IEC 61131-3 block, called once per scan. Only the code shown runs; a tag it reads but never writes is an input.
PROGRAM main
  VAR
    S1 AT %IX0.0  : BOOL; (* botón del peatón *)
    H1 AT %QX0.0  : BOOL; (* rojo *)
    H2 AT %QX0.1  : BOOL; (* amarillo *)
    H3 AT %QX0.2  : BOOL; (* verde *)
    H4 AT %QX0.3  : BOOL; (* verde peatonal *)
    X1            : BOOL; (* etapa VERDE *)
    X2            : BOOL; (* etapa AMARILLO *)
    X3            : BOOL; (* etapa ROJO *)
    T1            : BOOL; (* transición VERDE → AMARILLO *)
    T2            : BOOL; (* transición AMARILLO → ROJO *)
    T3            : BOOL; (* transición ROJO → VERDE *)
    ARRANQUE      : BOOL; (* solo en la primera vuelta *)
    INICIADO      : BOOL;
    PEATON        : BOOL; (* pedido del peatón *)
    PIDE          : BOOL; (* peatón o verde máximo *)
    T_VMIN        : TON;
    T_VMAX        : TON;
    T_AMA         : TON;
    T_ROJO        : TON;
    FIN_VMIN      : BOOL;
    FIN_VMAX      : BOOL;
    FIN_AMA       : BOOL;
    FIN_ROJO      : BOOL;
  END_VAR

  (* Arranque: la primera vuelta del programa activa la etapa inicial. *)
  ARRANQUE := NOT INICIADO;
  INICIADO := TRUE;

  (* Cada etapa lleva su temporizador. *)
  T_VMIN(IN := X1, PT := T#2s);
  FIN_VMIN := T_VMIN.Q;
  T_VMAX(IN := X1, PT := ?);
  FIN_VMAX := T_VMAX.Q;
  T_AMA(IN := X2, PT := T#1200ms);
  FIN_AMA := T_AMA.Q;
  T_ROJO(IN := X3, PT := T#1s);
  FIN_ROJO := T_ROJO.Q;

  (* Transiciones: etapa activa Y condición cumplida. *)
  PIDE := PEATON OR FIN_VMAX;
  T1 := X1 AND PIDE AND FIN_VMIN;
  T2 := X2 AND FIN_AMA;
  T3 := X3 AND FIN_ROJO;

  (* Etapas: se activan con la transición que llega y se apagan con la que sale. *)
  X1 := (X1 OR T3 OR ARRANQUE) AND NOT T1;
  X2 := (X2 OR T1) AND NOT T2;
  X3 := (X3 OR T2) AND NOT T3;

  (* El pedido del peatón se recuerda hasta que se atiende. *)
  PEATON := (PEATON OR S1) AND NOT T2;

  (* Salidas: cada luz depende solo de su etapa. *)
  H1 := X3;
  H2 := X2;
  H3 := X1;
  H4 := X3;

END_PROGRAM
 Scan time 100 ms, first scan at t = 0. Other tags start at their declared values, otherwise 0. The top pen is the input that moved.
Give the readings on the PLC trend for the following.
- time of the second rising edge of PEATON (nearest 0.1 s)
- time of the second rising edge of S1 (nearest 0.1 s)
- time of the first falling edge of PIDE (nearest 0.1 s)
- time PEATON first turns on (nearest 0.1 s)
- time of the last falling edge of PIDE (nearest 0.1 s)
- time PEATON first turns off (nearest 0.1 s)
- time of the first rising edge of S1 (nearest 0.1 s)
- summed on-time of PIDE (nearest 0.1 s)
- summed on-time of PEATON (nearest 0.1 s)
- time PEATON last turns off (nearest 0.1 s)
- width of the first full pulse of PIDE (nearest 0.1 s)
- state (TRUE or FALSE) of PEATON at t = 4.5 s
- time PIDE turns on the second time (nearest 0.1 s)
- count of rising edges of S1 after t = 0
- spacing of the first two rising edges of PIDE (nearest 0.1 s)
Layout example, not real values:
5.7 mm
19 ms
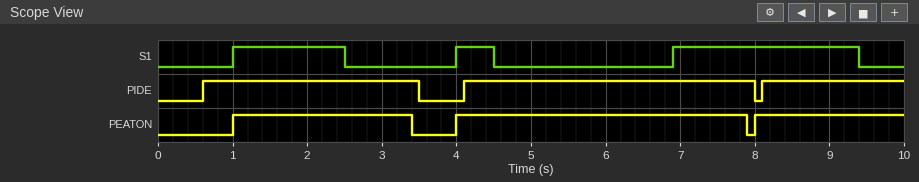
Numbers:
4.0 s
4.0 s
3.5 s
1.0 s
8.0 s
3.4 s
1.0 s
8.7 s
8.3 s
7.9 s
2.9 s
TRUE
4.1 s
3
3.5 s
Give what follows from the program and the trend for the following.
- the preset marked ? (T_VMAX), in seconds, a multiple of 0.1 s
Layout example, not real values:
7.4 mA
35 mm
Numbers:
0.5 s
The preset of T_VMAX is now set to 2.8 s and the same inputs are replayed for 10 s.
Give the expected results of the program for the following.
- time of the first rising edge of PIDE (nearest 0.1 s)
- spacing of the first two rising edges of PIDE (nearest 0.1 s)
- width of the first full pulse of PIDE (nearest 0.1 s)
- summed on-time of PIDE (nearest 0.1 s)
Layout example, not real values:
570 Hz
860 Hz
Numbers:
1.1 s
3.0 s
2.4 s
8.2 s
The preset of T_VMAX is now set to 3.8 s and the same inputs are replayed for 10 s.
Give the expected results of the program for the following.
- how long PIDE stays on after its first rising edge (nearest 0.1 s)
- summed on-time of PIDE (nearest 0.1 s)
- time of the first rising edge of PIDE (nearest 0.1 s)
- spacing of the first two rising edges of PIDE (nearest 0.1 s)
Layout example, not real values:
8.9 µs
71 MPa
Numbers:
2.4 s
8.2 s
1.1 s
3.0 s
